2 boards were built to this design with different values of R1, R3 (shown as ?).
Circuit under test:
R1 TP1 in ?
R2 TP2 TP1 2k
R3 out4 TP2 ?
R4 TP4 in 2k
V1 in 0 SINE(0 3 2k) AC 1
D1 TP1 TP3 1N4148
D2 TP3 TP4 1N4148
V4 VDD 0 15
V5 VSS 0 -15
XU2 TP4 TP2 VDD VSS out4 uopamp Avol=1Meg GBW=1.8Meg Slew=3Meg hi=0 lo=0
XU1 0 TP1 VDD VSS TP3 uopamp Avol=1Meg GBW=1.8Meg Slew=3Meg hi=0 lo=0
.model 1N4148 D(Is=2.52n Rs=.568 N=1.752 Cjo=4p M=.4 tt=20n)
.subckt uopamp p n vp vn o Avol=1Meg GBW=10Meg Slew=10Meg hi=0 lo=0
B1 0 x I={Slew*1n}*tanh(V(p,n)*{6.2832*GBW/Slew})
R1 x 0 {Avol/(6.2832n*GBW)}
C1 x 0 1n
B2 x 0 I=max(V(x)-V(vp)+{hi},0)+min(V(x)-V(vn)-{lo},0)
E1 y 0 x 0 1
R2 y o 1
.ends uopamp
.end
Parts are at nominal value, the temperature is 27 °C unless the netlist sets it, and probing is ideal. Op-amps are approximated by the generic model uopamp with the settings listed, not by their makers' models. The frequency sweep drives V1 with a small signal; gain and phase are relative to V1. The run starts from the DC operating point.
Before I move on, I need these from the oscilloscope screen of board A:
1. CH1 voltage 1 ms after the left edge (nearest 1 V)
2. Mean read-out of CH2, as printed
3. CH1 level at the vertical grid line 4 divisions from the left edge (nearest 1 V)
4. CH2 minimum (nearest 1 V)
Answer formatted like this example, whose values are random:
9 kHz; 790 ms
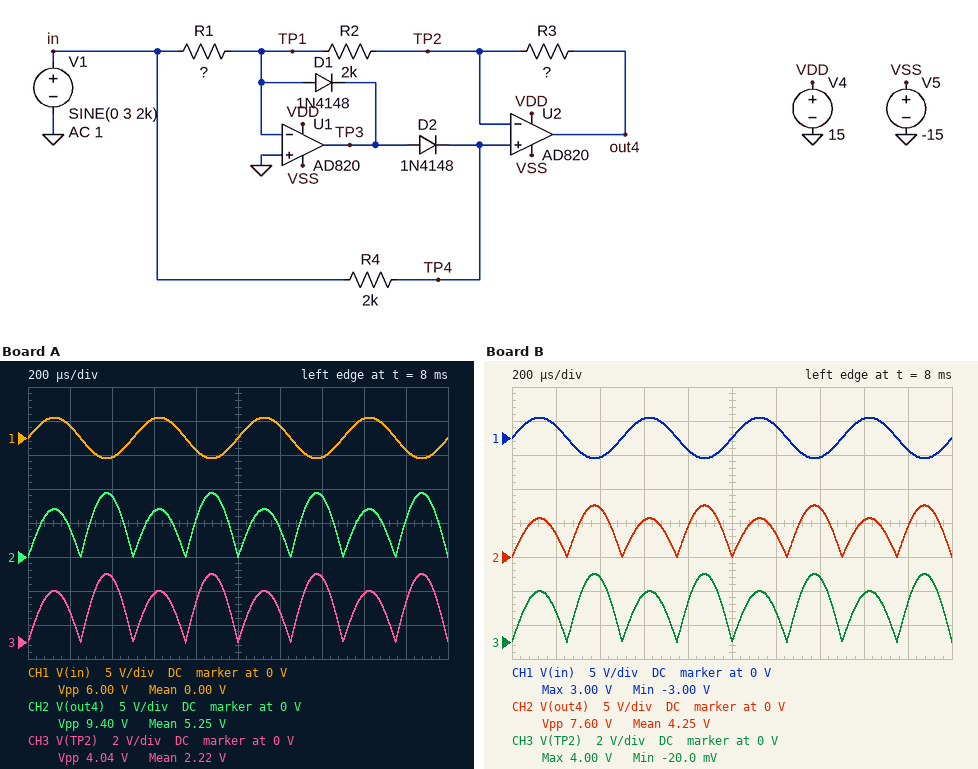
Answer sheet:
0 V; 5.25 V; -2 V; 0 V
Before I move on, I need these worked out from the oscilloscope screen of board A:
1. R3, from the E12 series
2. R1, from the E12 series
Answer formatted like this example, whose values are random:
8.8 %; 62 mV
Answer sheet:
2.7 kΩ; 1.5 kΩ
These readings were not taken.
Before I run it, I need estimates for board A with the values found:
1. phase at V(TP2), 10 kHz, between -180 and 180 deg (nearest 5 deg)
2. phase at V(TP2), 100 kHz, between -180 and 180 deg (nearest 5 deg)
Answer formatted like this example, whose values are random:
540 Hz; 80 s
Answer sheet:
0 deg; -5 deg
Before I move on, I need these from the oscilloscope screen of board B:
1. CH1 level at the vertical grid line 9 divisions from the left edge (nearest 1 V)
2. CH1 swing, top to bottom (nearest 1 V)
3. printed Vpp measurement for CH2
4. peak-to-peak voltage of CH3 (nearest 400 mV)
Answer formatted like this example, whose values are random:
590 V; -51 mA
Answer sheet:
-2 V; 6 V; 7.60 V; 4.0 V
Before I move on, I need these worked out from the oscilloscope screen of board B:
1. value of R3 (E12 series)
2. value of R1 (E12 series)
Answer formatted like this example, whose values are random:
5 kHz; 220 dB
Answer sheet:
1.8 kΩ; 1.5 kΩ
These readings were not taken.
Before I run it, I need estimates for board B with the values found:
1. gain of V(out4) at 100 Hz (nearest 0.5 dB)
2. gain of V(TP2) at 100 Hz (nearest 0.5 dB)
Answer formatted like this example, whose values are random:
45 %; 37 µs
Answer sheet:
-5.5 dB; -6.0 dB
